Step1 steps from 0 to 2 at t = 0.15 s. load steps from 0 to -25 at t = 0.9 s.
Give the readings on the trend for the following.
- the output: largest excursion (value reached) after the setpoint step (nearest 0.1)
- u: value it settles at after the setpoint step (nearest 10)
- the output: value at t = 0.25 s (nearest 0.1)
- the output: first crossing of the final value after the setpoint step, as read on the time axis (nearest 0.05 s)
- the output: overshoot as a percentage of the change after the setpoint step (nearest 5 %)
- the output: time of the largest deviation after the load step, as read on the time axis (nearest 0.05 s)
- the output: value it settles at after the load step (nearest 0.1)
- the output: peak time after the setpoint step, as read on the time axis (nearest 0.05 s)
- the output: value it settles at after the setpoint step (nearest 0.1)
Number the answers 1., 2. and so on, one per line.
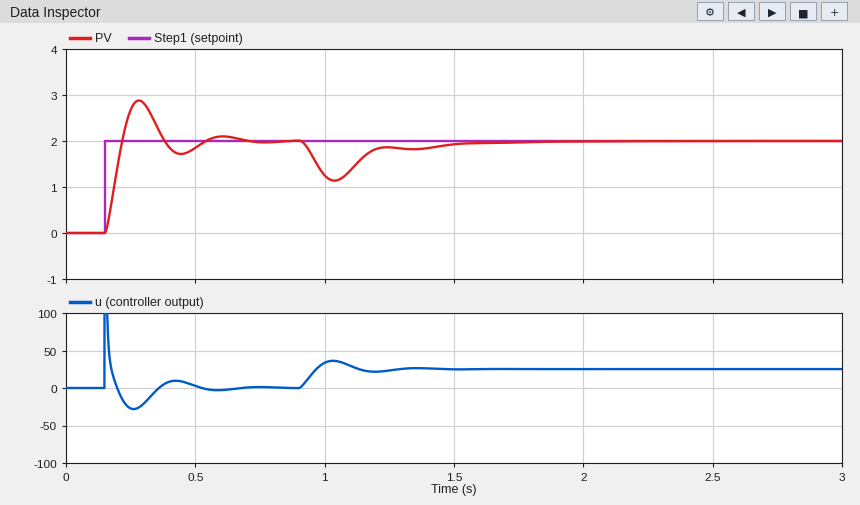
1. 2.9
2. 0
3. 2.7
4. 0.20 s
5. 45 %
6. 1.05 s
7. 2.0
8. 0.30 s
9. 2.0
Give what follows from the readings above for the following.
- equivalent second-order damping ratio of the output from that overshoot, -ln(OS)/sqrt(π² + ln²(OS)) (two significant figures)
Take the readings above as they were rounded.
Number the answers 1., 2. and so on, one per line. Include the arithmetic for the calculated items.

1. ln(0.45) = -0.799; 0.799 / sqrt(9.870 + 0.638) = 0.25
